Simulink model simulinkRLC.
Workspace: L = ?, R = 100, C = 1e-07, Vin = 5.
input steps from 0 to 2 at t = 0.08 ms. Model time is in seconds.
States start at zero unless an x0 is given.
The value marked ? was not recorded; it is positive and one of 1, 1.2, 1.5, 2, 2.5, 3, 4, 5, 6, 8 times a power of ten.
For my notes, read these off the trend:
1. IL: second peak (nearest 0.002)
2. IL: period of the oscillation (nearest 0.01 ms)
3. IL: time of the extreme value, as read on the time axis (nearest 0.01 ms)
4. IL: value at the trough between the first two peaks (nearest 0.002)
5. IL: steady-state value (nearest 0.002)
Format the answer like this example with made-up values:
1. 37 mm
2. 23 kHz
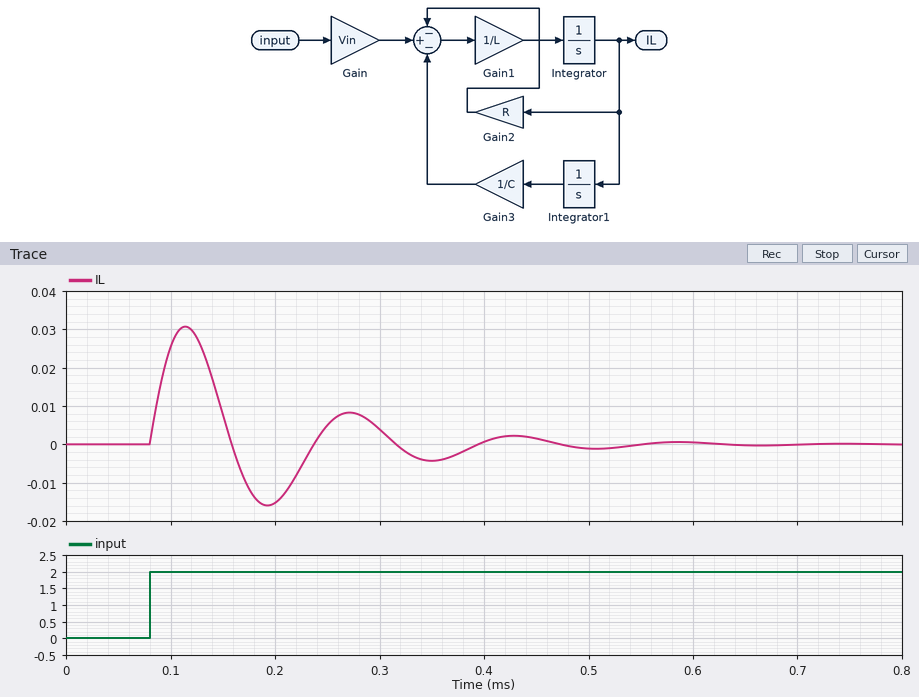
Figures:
1. 0.008
2. 0.16 ms
3. 0.11 ms
4. -0.016
5. 0.000
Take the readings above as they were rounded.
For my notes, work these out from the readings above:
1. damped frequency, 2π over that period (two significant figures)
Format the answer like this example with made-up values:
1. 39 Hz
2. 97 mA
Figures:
1. 39 rad/ms
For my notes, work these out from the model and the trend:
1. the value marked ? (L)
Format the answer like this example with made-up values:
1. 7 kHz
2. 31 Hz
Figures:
1. 0.006
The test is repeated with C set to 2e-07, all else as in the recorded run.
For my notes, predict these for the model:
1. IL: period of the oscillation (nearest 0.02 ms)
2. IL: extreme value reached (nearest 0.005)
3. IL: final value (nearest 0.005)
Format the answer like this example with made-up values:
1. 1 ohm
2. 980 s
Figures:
1. 0.22 ms
2. 0.040
3. 0.000
